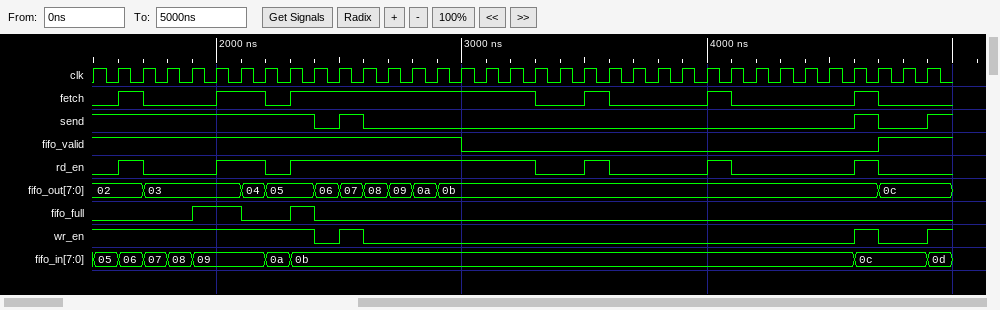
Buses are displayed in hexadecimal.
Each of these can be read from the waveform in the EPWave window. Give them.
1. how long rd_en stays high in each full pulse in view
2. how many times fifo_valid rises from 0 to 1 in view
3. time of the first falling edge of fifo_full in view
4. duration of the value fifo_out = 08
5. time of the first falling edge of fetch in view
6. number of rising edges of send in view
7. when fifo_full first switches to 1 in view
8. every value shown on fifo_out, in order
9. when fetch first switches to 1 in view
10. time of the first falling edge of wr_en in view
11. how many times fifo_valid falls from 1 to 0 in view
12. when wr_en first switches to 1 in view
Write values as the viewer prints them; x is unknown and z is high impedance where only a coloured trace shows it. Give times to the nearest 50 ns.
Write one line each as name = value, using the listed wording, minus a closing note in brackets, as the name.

how long rd_en stays high in each full pulse in view = 100 ns, 200 ns, 1000 ns, 100 ns, 100 ns, 100 ns
how many times fifo_valid rises from 0 to 1 in view = 1
time of the first falling edge of fifo_full in view = 2100 ns
duration of the value fifo_out = 08 = 100 ns
time of the first falling edge of fetch in view = 1700 ns
number of rising edges of send in view = 3
when fifo_full first switches to 1 in view = 1900 ns
every value shown on fifo_out, in order = 02, 03, 04, 05, 06, 07, 08, 09, 0a, 0b, 0c
when fetch first switches to 1 in view = 1600 ns
time of the first falling edge of wr_en in view = 2400 ns
how many times fifo_valid falls from 1 to 0 in view = 1
when wr_en first switches to 1 in view = 2500 ns
